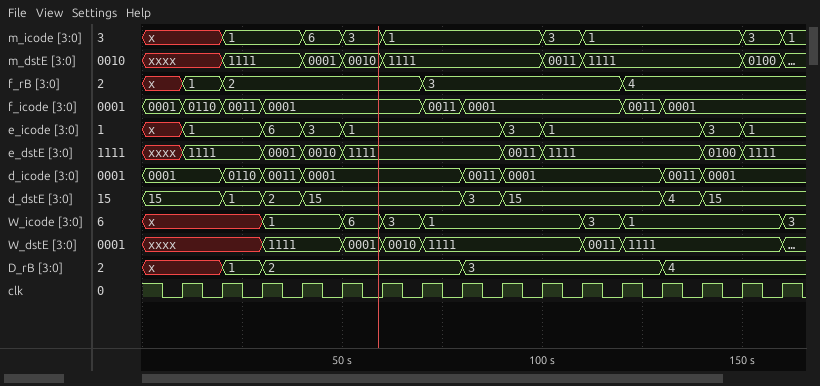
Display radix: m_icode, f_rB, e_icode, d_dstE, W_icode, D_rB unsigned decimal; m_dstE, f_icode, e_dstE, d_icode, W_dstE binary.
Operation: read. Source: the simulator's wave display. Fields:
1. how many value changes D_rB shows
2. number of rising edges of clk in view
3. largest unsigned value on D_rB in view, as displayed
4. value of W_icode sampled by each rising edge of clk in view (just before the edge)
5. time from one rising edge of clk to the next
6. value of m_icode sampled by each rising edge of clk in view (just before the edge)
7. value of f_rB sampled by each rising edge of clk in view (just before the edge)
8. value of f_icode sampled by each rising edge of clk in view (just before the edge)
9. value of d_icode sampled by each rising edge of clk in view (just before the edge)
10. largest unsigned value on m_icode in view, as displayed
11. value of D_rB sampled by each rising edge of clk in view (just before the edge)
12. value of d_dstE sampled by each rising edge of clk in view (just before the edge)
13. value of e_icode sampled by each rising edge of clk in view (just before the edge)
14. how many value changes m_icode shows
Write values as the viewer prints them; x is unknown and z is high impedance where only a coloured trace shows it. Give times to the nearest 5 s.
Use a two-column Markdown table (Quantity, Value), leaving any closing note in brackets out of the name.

| Quantity | Value |
|---|---|
| how many value changes D_rB shows | 4 |
| number of rising edges of clk in view | 16 |
| largest unsigned value on D_rB in view, as displayed | 4 |
| value of W_icode sampled by each rising edge of clk in view | x, x, x, 1, 1, 6, 3, 1, 1, 1, 1, 3, 1, 1, 1, 1 |
| time from one rising edge of clk to the next | 10 s |
| value of m_icode sampled by each rising edge of clk in view | x, x, 1, 1, 6, 3, 1, 1, 1, 1, 3, 1, 1, 1, 1, 3 |
| value of f_rB sampled by each rising edge of clk in view | x, 1, 2, 2, 2, 2, 2, 3, 3, 3, 3, 3, 4, 4, 4, 4 |
| value of f_icode sampled by each rising edge of clk in view | 0001, 0110, 0011, 0001, 0001, 0001, 0001, 0011, 0001, 0001, 0001, 0001, 0011, 0001, 0001, 0001 |
| value of d_icode sampled by each rising edge of clk in view | 0001, 0001, 0110, 0011, 0001, 0001, 0001, 0001, 0011, 0001, 0001, 0001, 0001, 0011, 0001, 0001 |
| largest unsigned value on m_icode in view, as displayed | 6 |
| value of D_rB sampled by each rising edge of clk in view | x, x, 1, 2, 2, 2, 2, 2, 3, 3, 3, 3, 3, 4, 4, 4 |
| value of d_dstE sampled by each rising edge of clk in view | 15, 15, 1, 2, 15, 15, 15, 15, 3, 15, 15, 15, 15, 4, 15, 15 |
| value of e_icode sampled by each rising edge of clk in view | x, 1, 1, 6, 3, 1, 1, 1, 1, 3, 1, 1, 1, 1, 3, 1 |
| how many value changes m_icode shows | 8 |
